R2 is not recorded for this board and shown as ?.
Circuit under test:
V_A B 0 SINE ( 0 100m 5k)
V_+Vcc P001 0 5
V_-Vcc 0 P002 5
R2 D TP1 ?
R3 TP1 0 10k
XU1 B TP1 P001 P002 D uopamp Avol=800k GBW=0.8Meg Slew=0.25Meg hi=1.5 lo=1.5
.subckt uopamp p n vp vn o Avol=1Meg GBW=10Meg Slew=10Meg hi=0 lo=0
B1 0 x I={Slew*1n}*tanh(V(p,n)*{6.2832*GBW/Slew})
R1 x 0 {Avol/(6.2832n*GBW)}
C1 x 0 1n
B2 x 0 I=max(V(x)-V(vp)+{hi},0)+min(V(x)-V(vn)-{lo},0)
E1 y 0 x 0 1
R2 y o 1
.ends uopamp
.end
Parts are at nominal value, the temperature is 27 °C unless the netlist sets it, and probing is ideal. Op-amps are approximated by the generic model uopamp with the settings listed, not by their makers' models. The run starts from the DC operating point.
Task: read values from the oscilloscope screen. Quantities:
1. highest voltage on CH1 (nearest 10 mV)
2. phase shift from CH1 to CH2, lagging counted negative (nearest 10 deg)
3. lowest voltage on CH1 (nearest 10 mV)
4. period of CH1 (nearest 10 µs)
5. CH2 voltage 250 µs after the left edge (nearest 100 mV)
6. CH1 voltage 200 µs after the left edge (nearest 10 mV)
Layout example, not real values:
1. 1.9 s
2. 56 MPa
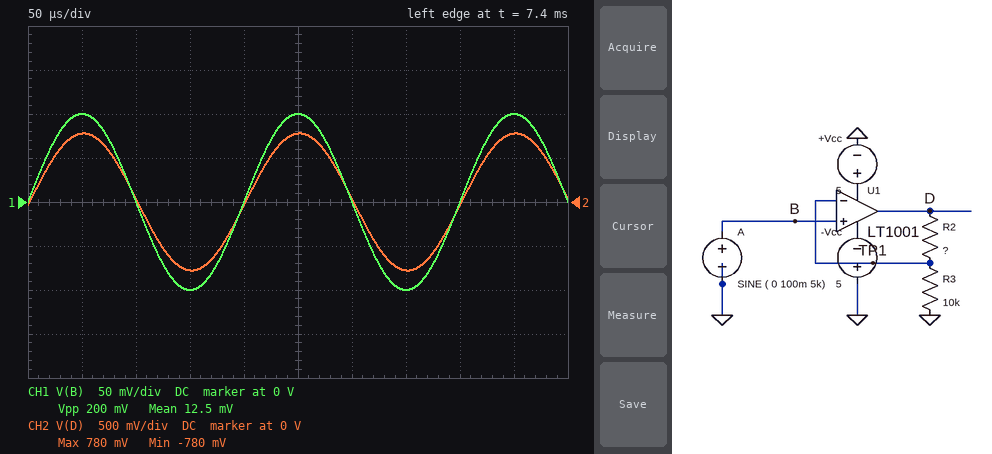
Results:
1. 100 mV
2. 0 deg
3. -100 mV
4. 200 µs
5. 800 mV
6. 0 V
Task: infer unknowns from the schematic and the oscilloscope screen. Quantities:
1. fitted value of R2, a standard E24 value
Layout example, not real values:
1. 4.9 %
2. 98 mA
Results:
1. 68 kΩ
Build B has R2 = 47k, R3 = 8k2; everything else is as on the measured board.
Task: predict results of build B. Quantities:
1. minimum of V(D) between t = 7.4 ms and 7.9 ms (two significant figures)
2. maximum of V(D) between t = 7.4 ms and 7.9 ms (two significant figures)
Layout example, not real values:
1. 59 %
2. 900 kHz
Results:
1. -670 mV
2. 670 mV
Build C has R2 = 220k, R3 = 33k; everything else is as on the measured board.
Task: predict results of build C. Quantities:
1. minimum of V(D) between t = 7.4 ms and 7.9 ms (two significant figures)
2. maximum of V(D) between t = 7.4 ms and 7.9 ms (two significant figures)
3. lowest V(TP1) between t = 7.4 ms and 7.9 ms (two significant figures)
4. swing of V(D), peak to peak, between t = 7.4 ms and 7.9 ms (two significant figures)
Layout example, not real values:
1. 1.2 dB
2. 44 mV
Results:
1. -770 mV
2. 770 mV
3. -100 mV
4. 1.5 V
